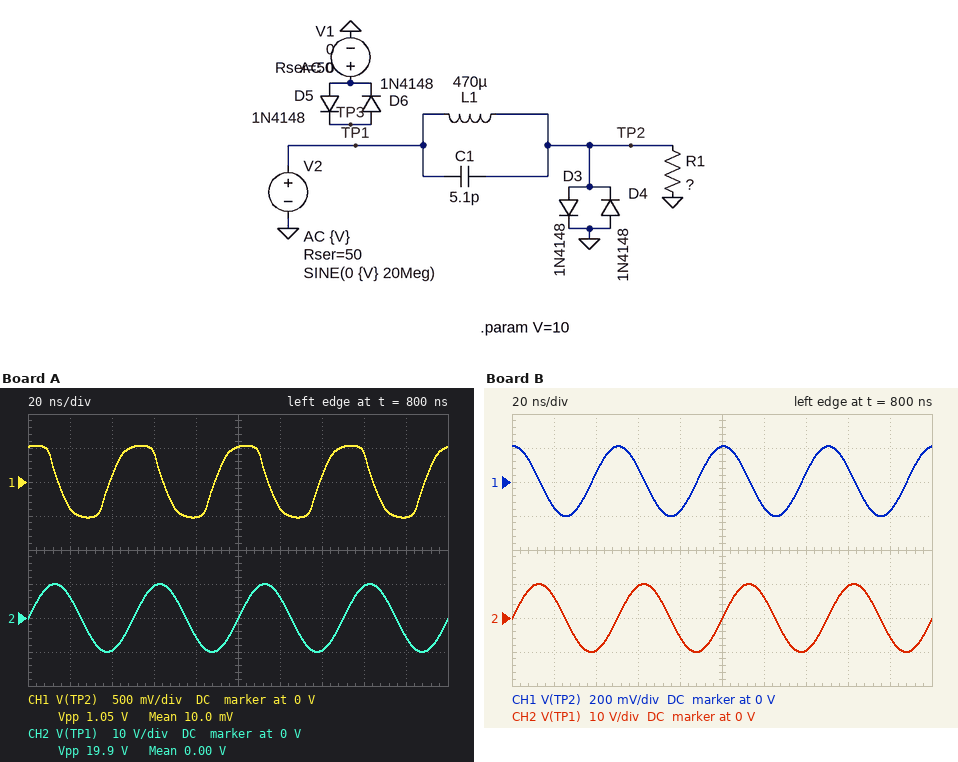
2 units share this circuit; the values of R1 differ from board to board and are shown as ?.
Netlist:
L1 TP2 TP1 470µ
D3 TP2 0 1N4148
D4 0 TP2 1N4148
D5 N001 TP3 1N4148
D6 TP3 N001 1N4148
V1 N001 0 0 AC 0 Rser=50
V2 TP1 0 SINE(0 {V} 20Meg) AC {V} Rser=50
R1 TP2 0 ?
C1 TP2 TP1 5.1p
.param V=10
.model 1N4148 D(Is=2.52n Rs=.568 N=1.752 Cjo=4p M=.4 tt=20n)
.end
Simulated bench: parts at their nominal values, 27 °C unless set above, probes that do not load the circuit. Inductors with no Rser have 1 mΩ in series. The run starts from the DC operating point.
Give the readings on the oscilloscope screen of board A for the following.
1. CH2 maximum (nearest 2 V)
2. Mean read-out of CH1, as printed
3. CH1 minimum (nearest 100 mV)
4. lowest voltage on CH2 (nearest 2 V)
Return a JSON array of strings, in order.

["10 V", "10.0 mV", "-500 mV", "-10 V"]
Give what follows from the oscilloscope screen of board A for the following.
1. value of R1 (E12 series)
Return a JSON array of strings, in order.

["100 Ω"]
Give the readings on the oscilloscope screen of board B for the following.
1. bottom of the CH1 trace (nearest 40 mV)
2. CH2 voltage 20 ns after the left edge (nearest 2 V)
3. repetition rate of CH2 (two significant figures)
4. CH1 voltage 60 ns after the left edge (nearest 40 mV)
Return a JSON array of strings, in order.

["-200 mV", "6 V", "20 MHz", "80 mV"]
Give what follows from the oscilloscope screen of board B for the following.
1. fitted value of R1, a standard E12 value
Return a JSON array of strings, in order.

["33 Ω"]
